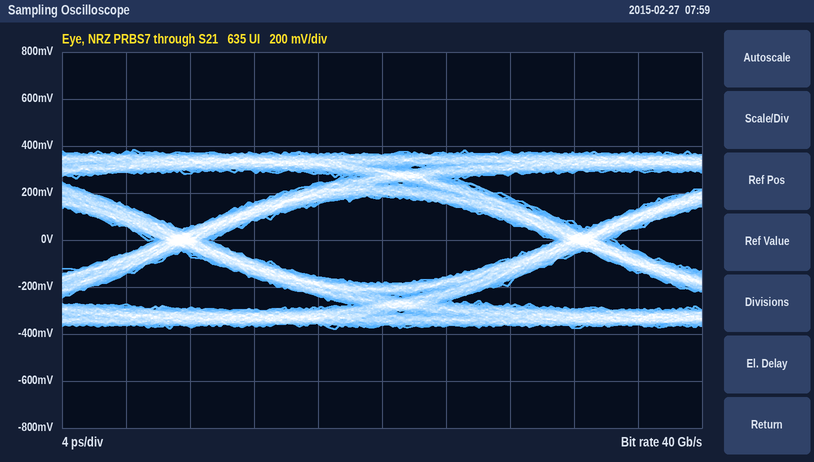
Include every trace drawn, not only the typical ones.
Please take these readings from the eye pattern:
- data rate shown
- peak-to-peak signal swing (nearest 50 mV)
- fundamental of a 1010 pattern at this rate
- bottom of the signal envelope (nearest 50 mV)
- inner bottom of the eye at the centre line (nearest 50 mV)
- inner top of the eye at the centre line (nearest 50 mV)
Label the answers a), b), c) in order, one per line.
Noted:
a) 40 Gb/s
b) 750 mV
c) 20 GHz
d) -400 mV
e) -200 mV
f) 200 mV
